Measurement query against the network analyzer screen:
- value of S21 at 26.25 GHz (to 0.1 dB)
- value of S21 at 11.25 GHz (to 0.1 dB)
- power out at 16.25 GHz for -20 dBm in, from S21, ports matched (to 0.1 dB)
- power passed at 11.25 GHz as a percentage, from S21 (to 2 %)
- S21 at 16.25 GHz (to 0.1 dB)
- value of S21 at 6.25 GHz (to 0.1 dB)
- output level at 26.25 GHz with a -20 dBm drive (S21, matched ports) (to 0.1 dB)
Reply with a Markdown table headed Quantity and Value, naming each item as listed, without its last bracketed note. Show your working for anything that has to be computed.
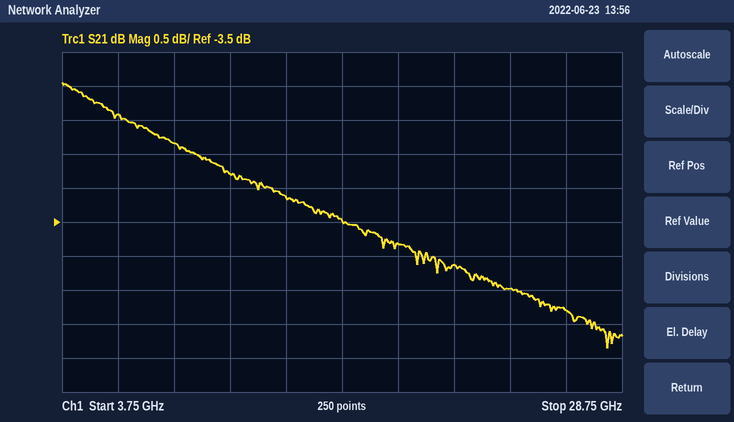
| Quantity | Value |
|---|---|
| value of S21 at 26.25 GHz | -4.8 dB |
| value of S21 at 11.25 GHz | -2.8 dB |
| power out at 16.25 GHz for -20 dBm in, from S21, ports matched | -20 dBm + (-3.5 dB) = -23.5 dBm |
| power passed at 11.25 GHz as a percentage, from S21 | 10^(-2.8/10) ≈ 52 % |
| S21 at 16.25 GHz | -3.5 dB |
| value of S21 at 6.25 GHz | -1.9 dB |
| output level at 26.25 GHz with a -20 dBm drive (S21, matched ports) | -20 dBm + (-4.8 dB) = -24.8 dBm |
